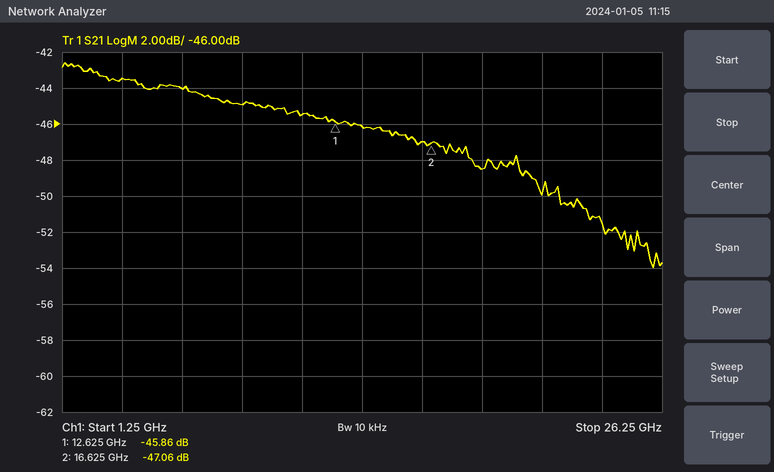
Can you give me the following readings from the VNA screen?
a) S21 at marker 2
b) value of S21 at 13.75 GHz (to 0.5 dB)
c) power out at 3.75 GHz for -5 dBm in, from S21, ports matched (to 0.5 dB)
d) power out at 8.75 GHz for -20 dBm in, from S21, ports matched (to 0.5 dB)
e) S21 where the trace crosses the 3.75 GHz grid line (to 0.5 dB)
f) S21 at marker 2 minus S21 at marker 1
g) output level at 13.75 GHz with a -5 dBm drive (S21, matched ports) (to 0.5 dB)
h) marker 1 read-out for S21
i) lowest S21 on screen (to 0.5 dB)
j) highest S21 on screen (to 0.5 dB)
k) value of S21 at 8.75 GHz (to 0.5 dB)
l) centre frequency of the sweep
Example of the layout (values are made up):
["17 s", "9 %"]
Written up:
["-47.06 dB", "-46.0 dB", "-48.5 dBm", "-65.0 dBm", "-43.5 dB", "-1.20 dB", "-51.0 dBm", "-45.86 dB", "-54.0 dB", "-42.5 dB", "-45.0 dB", "13.75 GHz"]
